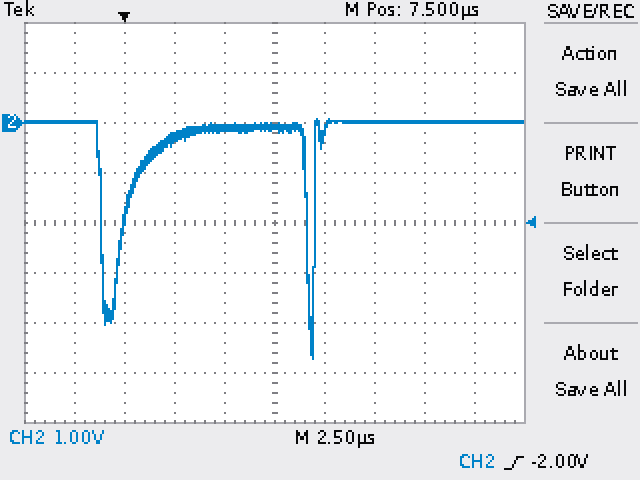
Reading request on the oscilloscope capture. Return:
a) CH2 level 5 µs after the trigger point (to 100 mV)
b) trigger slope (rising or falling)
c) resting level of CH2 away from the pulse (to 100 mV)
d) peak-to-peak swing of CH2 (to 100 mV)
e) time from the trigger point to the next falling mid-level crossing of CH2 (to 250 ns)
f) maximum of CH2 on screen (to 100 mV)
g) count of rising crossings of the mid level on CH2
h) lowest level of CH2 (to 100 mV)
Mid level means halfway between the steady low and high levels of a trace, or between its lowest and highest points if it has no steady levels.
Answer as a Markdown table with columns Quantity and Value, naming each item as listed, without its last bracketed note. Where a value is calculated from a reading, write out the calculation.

| Quantity | Value |
|---|---|
| CH2 level 5 µs after the trigger point | -100 mV |
| trigger slope | rising |
| resting level of CH2 away from the pulse | 0.0 V |
| peak-to-peak swing of CH2 | 100 mV − (-4.7 V) = 4.8 V |
| time from the trigger point to the next falling mid-level crossing of CH2 | 9.25 µs |
| maximum of CH2 on screen | 100 mV |
| count of rising crossings of the mid level on CH2 | 2 |
| lowest level of CH2 | -4.7 V |
